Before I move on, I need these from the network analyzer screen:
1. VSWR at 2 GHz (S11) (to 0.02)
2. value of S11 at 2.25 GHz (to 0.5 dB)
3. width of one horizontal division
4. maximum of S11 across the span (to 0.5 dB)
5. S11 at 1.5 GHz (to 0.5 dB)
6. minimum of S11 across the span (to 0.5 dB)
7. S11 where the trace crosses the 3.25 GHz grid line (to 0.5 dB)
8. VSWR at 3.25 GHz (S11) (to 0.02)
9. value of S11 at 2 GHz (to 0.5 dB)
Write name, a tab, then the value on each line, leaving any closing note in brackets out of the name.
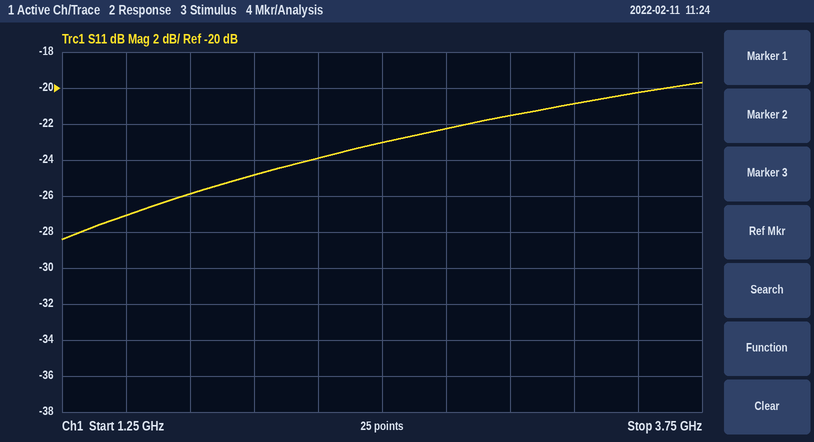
VSWR at 2 GHz (S11)	1.12
value of S11 at 2.25 GHz	-24.0 dB
width of one horizontal division	250 MHz
maximum of S11 across the span	-19.5 dB
S11 at 1.5 GHz	-27.0 dB
minimum of S11 across the span	-28.5 dB
S11 where the trace crosses the 3.25 GHz grid line	-21.0 dB
VSWR at 3.25 GHz (S11)	1.20
value of S11 at 2 GHz	-25.0 dB
